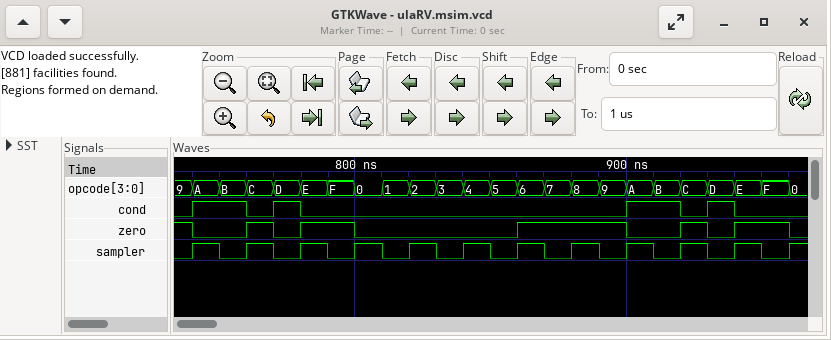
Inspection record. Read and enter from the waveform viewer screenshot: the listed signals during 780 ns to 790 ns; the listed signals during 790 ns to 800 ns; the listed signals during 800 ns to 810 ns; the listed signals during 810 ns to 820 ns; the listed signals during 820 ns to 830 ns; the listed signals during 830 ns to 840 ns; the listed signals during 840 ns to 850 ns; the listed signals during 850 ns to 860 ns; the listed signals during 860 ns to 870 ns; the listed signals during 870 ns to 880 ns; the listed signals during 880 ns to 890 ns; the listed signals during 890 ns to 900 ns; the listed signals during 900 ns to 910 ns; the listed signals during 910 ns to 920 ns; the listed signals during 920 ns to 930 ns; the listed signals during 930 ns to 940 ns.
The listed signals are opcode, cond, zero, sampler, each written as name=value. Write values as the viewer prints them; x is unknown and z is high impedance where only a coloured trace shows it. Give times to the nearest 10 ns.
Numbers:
opcode=E, cond=0, zero=1, sampler=1
opcode=F, cond=0, zero=1, sampler=0
opcode=0, cond=0, zero=0, sampler=1
opcode=1, cond=0, zero=0, sampler=0
opcode=2, cond=0, zero=0, sampler=1
opcode=3, cond=0, zero=0, sampler=0
opcode=4, cond=0, zero=0, sampler=1
opcode=5, cond=0, zero=0, sampler=0
opcode=6, cond=0, zero=1, sampler=1
opcode=7, cond=0, zero=1, sampler=0
opcode=8, cond=0, zero=1, sampler=1
opcode=9, cond=0, zero=1, sampler=0
opcode=A, cond=1, zero=0, sampler=1
opcode=B, cond=1, zero=0, sampler=0
opcode=C, cond=0, zero=1, sampler=1
opcode=D, cond=1, zero=0, sampler=0
